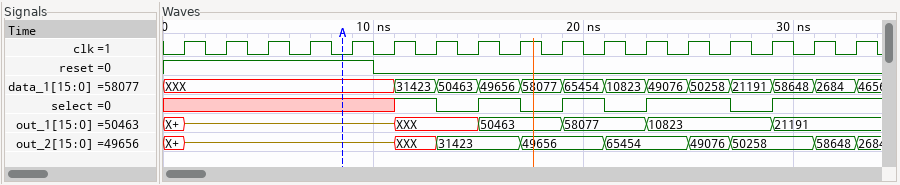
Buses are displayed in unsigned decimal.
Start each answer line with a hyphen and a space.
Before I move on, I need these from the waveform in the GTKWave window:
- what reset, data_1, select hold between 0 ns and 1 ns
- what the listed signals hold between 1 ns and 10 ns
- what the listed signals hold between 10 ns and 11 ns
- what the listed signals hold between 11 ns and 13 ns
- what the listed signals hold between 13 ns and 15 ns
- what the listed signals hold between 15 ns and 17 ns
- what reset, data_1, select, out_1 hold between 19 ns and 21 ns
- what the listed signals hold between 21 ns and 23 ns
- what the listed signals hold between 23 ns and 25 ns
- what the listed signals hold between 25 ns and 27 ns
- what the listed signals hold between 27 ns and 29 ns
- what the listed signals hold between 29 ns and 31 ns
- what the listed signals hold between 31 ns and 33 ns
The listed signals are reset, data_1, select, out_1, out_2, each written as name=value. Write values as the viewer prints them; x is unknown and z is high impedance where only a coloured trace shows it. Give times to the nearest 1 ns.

- reset=1, data_1=XXX, select=x
- reset=1, data_1=XXX, select=x, out_1=z, out_2=z
- reset=0, data_1=XXX, select=x, out_1=z, out_2=z
- reset=0, data_1=31423, select=1, out_1=XXX, out_2=XXX
- reset=0, data_1=50463, select=0, out_1=XXX, out_2=31423
- reset=0, data_1=49656, select=1, out_1=50463, out_2=31423
- reset=0, data_1=65454, select=1, out_1=58077
- reset=0, data_1=10823, select=0, out_1=58077, out_2=65454
- reset=0, data_1=49076, select=1, out_1=10823, out_2=65454
- reset=0, data_1=50258, select=1, out_1=10823, out_2=49076
- reset=0, data_1=21191, select=0, out_1=10823, out_2=50258
- reset=0, data_1=58648, select=1, out_1=21191, out_2=50258
- reset=0, data_1=2684, select=1, out_1=21191, out_2=58648
